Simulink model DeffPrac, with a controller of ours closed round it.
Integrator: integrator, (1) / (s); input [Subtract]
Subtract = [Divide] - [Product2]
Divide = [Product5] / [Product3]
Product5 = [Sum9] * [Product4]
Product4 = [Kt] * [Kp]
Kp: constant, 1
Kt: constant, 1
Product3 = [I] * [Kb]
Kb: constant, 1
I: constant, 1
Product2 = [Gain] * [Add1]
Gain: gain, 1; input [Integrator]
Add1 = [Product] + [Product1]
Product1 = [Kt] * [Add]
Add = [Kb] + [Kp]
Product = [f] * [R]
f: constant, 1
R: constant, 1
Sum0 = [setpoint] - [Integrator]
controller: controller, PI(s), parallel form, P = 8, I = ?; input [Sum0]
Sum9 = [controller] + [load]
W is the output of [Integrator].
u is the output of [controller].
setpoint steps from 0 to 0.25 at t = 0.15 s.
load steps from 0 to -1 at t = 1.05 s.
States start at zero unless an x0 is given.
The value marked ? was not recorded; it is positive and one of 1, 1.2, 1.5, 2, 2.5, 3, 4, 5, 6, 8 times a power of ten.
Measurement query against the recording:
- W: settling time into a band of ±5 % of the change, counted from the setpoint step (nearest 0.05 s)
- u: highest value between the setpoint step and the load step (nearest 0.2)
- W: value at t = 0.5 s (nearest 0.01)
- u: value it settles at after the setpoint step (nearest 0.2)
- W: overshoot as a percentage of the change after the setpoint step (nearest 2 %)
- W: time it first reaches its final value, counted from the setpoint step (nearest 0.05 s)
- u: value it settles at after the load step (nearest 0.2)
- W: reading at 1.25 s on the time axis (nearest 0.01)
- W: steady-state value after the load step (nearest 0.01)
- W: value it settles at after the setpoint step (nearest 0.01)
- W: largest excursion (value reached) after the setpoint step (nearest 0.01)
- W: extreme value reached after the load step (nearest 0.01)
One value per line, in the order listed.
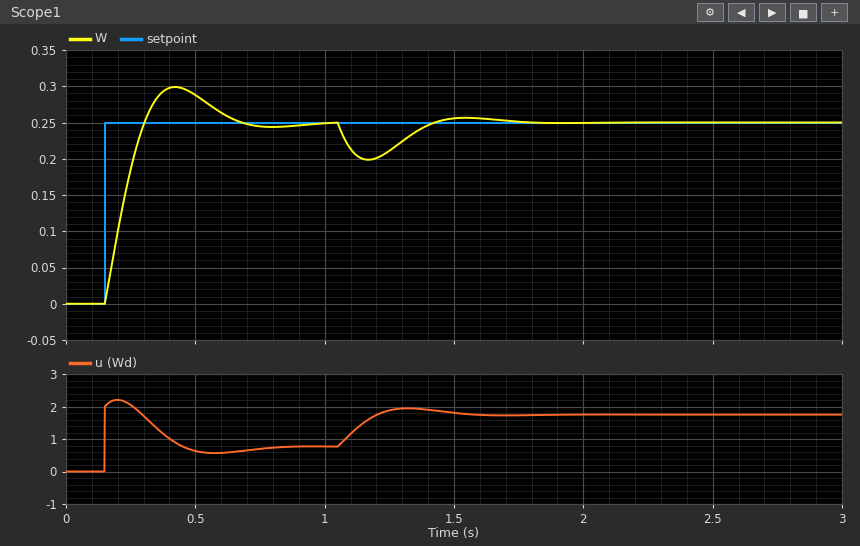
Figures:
0.45 s
2.2
0.29
0.8
20 %
0.15 s
1.8
0.21
0.25
0.25
0.30
0.20
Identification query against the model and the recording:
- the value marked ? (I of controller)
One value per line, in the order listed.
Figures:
100
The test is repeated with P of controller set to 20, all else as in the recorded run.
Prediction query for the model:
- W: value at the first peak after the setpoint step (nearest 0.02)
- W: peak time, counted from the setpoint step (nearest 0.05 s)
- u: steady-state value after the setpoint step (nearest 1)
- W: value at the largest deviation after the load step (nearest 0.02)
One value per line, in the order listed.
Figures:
0.26
0.25 s
1
0.22
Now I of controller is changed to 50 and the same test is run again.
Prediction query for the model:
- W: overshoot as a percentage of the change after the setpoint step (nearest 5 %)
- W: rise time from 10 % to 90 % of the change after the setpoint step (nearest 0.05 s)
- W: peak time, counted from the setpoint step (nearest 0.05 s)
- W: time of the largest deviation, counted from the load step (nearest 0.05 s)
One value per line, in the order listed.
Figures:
10 %
0.15 s
0.40 s
0.15 s
